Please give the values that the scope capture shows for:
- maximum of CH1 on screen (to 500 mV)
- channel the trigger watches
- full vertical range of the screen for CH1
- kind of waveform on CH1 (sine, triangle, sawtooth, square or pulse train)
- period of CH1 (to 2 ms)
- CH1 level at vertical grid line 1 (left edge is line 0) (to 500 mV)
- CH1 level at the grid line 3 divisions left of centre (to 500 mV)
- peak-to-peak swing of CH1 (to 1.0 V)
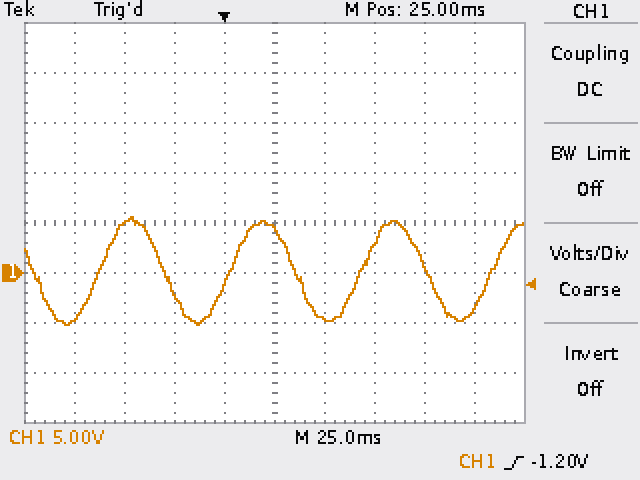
5.5 V
CH1
40 V
sine
66 ms
-4.5 V
5.0 V
11.0 V
